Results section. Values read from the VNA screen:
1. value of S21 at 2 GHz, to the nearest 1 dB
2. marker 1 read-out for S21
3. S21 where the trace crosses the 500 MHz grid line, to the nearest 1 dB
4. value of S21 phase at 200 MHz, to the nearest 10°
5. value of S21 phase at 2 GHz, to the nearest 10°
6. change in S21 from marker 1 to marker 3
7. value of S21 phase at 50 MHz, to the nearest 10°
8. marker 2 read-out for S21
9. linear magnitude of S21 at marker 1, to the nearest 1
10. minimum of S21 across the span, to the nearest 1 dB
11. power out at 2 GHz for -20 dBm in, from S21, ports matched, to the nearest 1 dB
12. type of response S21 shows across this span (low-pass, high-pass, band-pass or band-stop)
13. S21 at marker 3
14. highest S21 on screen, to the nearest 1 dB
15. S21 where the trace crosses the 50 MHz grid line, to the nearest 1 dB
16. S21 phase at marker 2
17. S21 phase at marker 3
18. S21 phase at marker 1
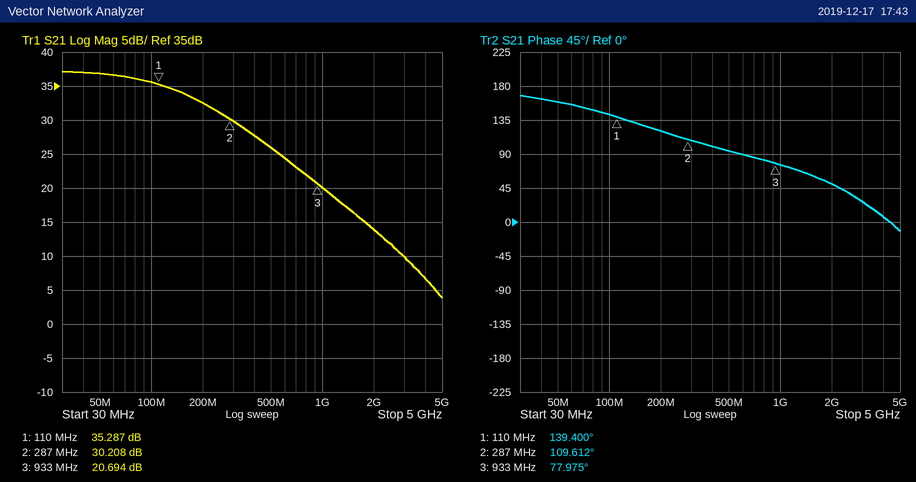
14 dB
35.287 dB
26 dB
120°
50°
-14.593 dB
160°
30.208 dB
58
4 dB
-6 dBm
low-pass
20.694 dB
37 dB
37 dB
109.612°
77.975°
139.400°
